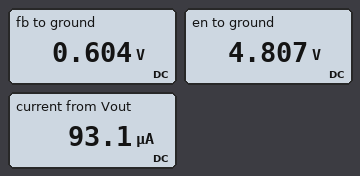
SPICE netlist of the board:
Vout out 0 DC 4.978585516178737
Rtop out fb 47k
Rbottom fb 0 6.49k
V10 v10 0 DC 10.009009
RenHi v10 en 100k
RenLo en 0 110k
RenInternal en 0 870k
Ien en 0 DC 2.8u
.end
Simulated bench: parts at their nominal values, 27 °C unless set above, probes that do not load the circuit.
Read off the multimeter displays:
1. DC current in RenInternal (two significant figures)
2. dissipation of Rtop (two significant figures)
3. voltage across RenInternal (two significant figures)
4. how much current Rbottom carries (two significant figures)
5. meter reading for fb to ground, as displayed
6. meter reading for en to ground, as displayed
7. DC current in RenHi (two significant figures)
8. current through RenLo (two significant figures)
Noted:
5.5 µA
410 µW
4.8 V
93 µA
0.604 V
4.807 V
52 µA
44 µA
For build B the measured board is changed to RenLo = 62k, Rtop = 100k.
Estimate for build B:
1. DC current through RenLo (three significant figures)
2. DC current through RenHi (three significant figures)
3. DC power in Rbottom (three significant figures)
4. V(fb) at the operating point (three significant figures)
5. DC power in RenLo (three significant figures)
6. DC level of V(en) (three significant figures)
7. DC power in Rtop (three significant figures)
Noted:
57.5 µA
64.4 µA
14.2 µW
303 mV
205 µW
3.57 V
219 µW
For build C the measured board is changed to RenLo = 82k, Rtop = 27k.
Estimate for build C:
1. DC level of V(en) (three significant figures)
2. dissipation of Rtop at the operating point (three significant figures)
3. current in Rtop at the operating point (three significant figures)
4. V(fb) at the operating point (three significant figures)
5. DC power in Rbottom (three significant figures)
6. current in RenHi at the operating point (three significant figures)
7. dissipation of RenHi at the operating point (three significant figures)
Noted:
4.17 V
597 µW
149 µA
965 mV
143 µW
58.4 µA
341 µW
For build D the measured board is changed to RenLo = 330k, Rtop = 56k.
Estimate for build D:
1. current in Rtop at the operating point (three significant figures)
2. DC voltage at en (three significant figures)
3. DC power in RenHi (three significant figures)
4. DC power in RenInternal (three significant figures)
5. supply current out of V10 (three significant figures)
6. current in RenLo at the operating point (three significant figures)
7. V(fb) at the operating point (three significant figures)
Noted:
79.7 µA
6.86 V
99.1 µW
54.1 µW
31.5 µA
20.8 µA
517 mV
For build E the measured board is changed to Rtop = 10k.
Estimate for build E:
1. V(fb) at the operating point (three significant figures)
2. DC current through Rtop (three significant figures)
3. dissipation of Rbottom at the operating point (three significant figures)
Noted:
1.96 V
302 µA
592 µW
